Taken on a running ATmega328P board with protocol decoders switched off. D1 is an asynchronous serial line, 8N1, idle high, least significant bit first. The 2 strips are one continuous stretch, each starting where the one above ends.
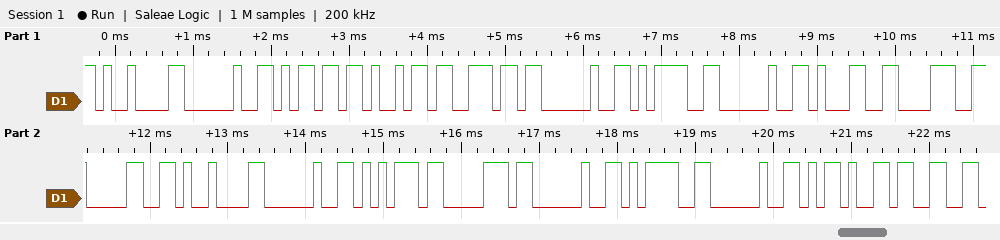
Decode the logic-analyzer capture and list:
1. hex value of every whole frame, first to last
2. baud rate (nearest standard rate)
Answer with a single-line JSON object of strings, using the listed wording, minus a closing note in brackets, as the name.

{"hex value of every whole frame, first to last": "0x09 0x20 0x6D 0x69 0x6E 0x20 0x3D 0x20 0x31 0x38 0x30 0x09 0x20 0x75 0x70 0x20 0x3D 0x20 0x2D 0x33", "baud rate": "9600 baud"}
